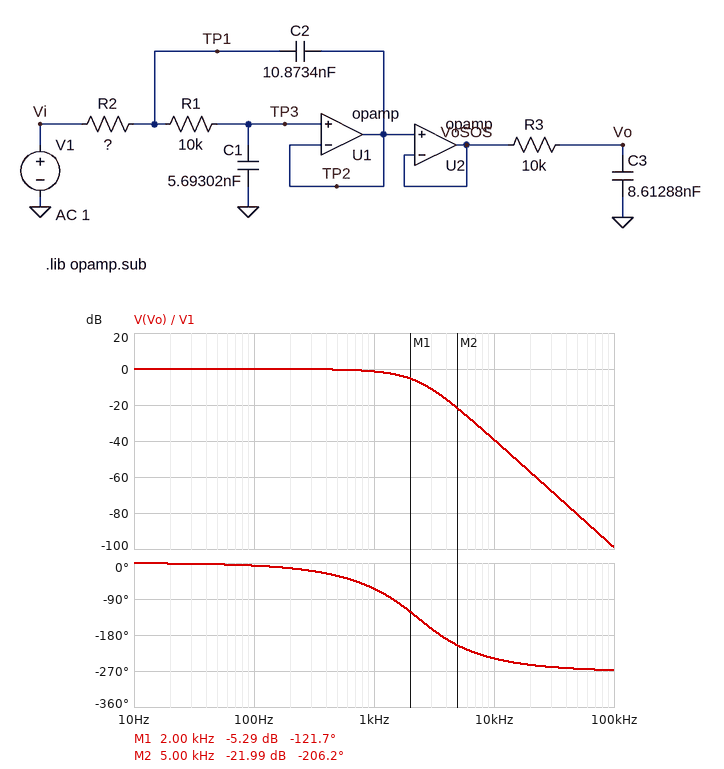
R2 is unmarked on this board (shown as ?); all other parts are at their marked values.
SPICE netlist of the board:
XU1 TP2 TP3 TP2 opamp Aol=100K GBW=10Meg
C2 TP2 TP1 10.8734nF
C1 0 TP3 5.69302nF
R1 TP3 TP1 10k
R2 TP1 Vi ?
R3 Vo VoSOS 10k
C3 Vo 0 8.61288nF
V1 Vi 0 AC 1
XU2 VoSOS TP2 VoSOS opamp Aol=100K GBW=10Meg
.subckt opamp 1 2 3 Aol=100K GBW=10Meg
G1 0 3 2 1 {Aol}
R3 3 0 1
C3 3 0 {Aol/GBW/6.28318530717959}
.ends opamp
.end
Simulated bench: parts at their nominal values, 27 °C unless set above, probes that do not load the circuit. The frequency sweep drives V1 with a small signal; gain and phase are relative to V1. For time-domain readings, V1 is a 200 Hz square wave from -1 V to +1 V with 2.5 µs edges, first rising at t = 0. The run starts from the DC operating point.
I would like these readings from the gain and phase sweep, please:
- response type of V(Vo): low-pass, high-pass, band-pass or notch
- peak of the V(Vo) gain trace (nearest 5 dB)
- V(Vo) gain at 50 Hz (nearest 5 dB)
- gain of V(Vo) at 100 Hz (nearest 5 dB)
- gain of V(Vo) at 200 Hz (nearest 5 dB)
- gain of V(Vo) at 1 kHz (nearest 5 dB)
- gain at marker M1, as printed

low-pass
0 dB
0 dB
0 dB
0 dB
0 dB
-5.29 dB
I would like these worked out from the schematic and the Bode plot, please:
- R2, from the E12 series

6.8 kΩ
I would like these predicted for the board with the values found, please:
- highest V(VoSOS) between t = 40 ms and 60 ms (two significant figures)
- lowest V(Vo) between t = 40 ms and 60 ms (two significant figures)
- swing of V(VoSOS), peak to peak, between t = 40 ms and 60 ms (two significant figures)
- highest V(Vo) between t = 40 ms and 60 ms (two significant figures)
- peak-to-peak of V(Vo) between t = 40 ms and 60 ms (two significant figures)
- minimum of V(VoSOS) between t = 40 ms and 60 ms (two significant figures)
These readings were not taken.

1.1 V
-1.0 V
2.1 V
1.0 V
2.0 V
-1.1 V
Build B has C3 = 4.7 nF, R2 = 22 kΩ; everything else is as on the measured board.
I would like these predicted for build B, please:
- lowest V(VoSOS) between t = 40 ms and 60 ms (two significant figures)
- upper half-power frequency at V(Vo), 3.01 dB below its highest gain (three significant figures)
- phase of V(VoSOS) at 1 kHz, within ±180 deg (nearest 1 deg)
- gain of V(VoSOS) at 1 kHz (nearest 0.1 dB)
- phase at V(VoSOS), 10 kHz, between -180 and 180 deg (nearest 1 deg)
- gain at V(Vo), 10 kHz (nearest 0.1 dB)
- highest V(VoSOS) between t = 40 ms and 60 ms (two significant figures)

-1.0 V
1.14 kHz
-68 deg
-1.8 dB
-168 deg
-44.5 dB
1.0 V
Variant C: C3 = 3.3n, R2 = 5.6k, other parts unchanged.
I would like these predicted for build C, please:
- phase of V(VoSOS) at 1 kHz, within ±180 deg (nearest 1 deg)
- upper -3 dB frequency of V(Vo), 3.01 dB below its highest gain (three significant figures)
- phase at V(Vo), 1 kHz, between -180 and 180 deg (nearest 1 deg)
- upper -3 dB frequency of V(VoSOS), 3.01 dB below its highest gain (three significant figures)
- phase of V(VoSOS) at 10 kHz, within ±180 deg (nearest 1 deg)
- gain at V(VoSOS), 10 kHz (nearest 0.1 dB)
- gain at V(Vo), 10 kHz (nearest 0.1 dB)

-33 deg
2.23 kHz
-45 deg
2.52 kHz
-156 deg
-22.8 dB
-30.1 dB
